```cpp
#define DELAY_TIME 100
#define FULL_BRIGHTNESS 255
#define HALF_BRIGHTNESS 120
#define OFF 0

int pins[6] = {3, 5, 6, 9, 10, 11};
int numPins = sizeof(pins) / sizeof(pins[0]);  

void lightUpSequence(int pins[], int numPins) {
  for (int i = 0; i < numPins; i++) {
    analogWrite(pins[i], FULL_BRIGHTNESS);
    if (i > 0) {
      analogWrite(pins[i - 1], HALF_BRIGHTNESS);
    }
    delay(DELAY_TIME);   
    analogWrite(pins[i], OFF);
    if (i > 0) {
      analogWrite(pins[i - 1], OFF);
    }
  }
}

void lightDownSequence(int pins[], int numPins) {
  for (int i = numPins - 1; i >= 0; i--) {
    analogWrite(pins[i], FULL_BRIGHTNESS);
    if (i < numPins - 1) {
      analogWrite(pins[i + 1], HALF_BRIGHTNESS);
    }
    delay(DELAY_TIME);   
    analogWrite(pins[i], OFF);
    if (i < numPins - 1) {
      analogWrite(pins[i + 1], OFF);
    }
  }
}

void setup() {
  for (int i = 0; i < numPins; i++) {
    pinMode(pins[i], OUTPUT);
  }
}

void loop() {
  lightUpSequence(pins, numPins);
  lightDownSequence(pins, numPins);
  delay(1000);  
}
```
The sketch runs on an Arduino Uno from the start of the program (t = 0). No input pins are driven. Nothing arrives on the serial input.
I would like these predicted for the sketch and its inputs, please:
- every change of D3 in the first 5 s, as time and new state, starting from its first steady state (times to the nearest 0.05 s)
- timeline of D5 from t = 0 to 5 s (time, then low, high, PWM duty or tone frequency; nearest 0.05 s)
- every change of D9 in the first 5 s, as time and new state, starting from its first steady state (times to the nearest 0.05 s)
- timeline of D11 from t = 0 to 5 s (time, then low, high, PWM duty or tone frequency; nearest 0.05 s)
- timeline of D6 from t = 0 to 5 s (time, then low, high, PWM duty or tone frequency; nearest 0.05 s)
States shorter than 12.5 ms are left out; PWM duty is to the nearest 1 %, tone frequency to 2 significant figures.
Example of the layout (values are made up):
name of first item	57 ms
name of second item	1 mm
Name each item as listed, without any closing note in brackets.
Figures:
every change of D3 in the first 5 s, as time and new state, starting from its first steady state	0 s high; 0.1 s PWM 47 %; 0.2 s low; 1.1 s high; 1.2 s low; 2.2 s high; 2.3 s PWM 47 %; 2.4 s low; 3.3 s high; 3.4 s low; 4.4 s high; 4.5 s PWM 47 %; 4.6 s low
timeline of D5 from t = 0 to 5 s	0 s low; 0.1 s high; 0.2 s PWM 47 %; 0.3 s low; 1 s high; 1.1 s PWM 47 %; 1.2 s low; 2.3 s high; 2.4 s PWM 47 %; 2.5 s low; 3.2 s high; 3.3 s PWM 47 %; 3.4 s low; 4.5 s high; 4.6 s PWM 47 %; 4.7 s low
every change of D9 in the first 5 s, as time and new state, starting from its first steady state	0 s low; 0.3 s high; 0.4 s PWM 47 %; 0.5 s low; 0.8 s high; 0.9 s PWM 47 %; 1 s low; 2.5 s high; 2.6 s PWM 47 %; 2.7 s low; 3 s high; 3.1 s PWM 47 %; 3.2 s low; 4.7 s high; 4.8 s PWM 47 %; 4.9 s low
timeline of D11 from t = 0 to 5 s	0 s low; 0.5 s high; 0.7 s PWM 47 %; 0.8 s low; 2.7 s high; 2.9 s PWM 47 %; 3 s low; 4.9 s high
timeline of D6 from t = 0 to 5 s	0 s low; 0.2 s high; 0.3 s PWM 47 %; 0.4 s low; 0.9 s high; 1 s PWM 47 %; 1.1 s low; 2.4 s high; 2.5 s PWM 47 %; 2.6 s low; 3.1 s high; 3.2 s PWM 47 %; 3.3 s low; 4.6 s high; 4.7 s PWM 47 %; 4.8 s low
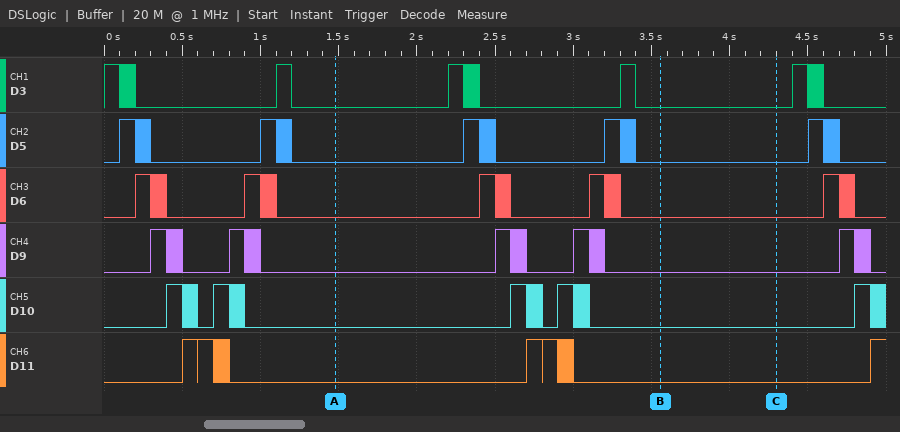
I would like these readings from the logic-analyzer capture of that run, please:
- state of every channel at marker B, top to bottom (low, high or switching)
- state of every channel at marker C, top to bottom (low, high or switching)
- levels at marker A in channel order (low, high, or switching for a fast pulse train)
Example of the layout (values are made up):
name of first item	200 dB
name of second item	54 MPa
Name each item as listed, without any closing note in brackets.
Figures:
state of every channel at marker B, top to bottom	D3 low, D5 low, D6 low, D9 low, D10 low, D11 low
state of every channel at marker C, top to bottom	D3 low, D5 low, D6 low, D9 low, D10 low, D11 low
levels at marker A in channel order	D3 low, D5 low, D6 low, D9 low, D10 low, D11 low
